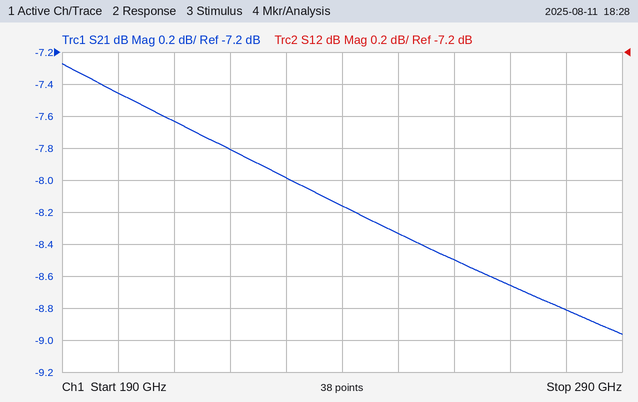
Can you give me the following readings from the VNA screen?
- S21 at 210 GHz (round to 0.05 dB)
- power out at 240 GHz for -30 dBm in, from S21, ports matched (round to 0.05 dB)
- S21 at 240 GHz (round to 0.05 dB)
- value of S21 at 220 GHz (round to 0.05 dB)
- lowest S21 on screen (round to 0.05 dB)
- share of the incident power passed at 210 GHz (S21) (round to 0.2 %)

-7.65 dB
-38.15 dBm
-8.15 dB
-7.80 dB
-8.95 dB
17.2 %
